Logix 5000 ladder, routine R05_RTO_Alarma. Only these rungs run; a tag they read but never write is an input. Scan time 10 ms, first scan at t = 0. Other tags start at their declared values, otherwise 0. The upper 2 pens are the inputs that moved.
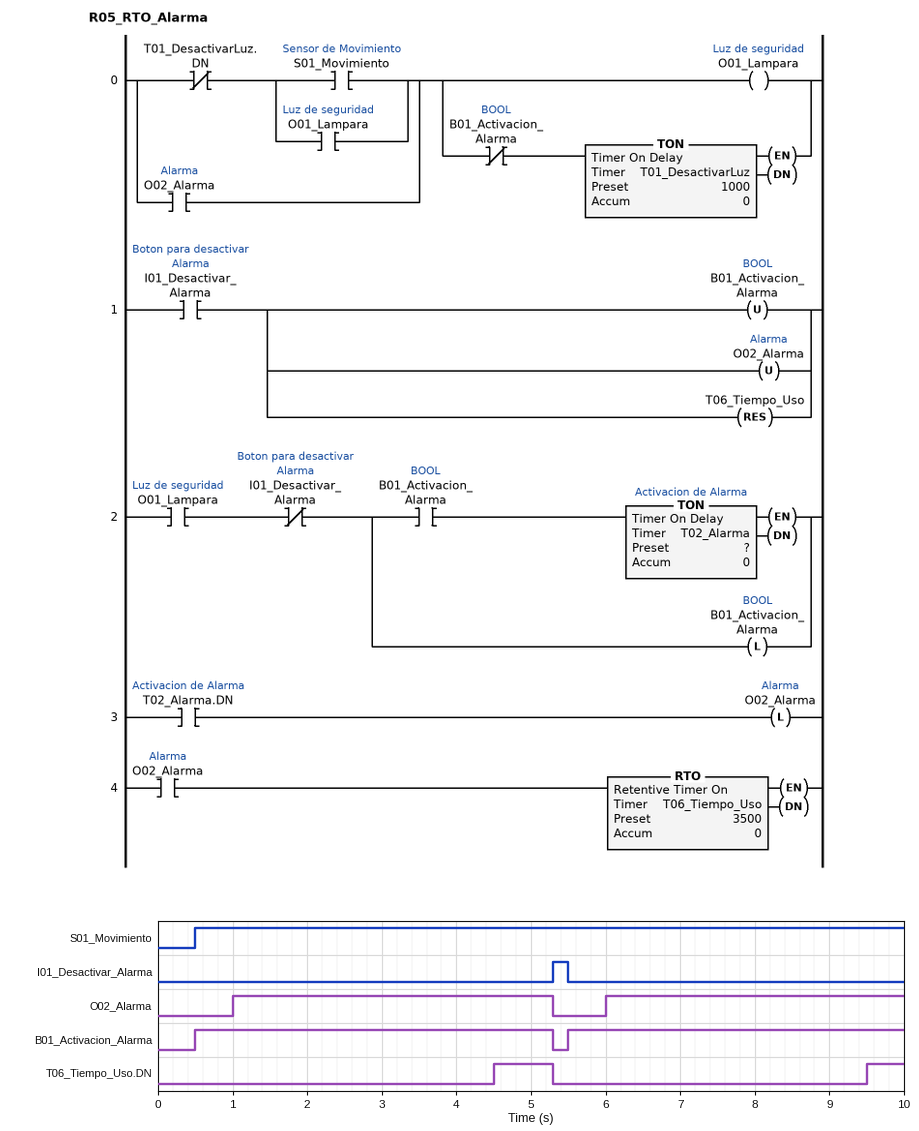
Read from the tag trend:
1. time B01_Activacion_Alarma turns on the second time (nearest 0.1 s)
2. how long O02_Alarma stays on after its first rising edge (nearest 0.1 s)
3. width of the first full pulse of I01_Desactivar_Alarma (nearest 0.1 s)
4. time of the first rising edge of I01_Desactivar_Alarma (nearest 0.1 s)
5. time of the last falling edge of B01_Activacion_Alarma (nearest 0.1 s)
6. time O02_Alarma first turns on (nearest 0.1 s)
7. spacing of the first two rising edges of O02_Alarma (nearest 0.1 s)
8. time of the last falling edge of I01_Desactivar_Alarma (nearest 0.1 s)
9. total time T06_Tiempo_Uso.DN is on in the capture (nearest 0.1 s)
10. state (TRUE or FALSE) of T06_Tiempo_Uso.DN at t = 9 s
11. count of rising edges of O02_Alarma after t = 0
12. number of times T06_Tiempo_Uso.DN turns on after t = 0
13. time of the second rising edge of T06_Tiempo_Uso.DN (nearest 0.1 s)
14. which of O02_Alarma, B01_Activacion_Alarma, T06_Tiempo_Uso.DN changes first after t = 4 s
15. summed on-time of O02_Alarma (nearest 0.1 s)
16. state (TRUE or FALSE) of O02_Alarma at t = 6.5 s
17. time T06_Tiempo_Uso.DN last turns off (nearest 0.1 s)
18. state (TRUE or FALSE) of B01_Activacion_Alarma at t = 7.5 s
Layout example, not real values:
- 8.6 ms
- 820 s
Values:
- 5.5 s
- 4.3 s
- 0.2 s
- 5.3 s
- 5.3 s
- 1.0 s
- 5.0 s
- 5.5 s
- 1.3 s
- FALSE
- 2
- 2
- 9.5 s
- T06_Tiempo_Uso.DN
- 8.3 s
- TRUE
- 5.3 s
- TRUE
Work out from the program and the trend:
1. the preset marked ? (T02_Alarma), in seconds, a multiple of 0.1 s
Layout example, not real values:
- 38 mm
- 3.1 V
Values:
- 0.5 s
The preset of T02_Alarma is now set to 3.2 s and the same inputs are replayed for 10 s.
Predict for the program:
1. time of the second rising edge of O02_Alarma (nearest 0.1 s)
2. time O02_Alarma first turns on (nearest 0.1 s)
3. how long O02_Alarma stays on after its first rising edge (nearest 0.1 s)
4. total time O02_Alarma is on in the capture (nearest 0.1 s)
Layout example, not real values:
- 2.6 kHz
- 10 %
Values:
- 8.7 s
- 3.7 s
- 1.6 s
- 2.9 s
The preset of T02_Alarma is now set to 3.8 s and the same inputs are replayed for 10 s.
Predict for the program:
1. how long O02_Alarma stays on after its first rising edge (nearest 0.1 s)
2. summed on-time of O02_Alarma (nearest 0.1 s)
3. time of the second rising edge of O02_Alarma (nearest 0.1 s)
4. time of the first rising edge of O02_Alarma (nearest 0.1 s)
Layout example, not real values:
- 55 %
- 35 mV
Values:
- 1.0 s
- 1.7 s
- 9.3 s
- 4.3 s
